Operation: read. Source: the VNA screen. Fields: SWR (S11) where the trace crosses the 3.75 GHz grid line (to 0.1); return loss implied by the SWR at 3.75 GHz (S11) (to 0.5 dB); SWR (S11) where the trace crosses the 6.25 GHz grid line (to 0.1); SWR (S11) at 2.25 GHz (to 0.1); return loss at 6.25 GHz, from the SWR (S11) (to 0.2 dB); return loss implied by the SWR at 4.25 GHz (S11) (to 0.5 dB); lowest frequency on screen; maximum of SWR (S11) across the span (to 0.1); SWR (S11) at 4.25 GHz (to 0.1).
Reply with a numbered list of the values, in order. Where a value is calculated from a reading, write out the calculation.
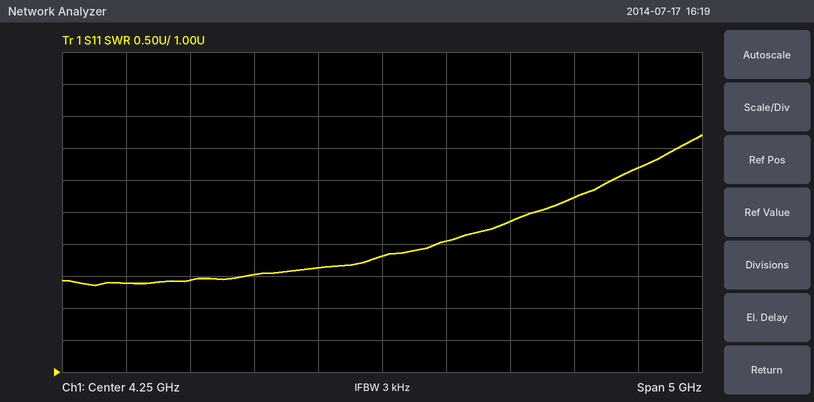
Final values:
1. 2.6
2. −20 log10((2.6 − 1)/(2.6 + 1)) ≈ 7.0 dB
3. 4.2
4. 2.4
5. −20 log10((4.2 − 1)/(4.2 + 1)) ≈ 4.2 dB
6. −20 log10((2.8 − 1)/(2.8 + 1)) ≈ 6.5 dB
7. 1.75 GHz
8. 4.7
9. 2.8
